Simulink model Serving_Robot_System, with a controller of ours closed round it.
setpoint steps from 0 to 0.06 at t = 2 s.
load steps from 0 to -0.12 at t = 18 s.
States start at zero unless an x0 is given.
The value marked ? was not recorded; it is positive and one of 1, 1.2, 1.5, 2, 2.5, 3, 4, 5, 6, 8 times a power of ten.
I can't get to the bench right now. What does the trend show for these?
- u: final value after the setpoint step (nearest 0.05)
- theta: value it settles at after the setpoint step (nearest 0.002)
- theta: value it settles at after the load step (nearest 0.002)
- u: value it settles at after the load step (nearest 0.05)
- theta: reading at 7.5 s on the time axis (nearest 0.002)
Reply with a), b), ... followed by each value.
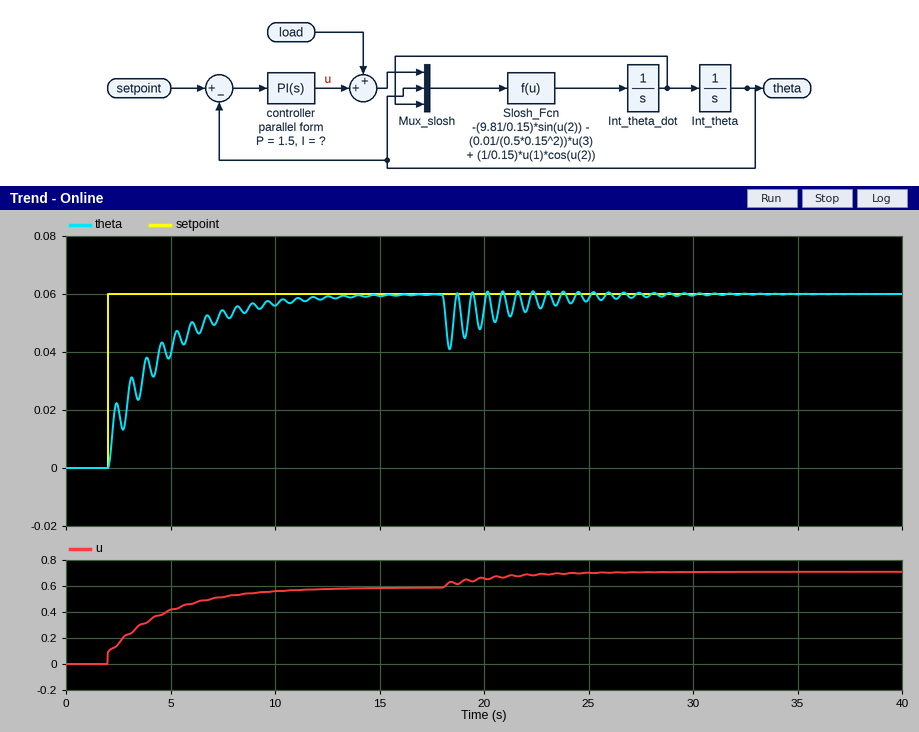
a) 0.60
b) 0.060
c) 0.060
d) 0.70
e) 0.054
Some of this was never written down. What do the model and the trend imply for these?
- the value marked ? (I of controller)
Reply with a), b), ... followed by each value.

a) 4
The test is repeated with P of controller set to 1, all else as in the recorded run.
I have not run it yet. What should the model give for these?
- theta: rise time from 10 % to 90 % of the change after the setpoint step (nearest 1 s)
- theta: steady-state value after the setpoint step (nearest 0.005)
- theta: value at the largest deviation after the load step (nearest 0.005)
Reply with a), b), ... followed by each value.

a) 5 s
b) 0.060
c) 0.040
